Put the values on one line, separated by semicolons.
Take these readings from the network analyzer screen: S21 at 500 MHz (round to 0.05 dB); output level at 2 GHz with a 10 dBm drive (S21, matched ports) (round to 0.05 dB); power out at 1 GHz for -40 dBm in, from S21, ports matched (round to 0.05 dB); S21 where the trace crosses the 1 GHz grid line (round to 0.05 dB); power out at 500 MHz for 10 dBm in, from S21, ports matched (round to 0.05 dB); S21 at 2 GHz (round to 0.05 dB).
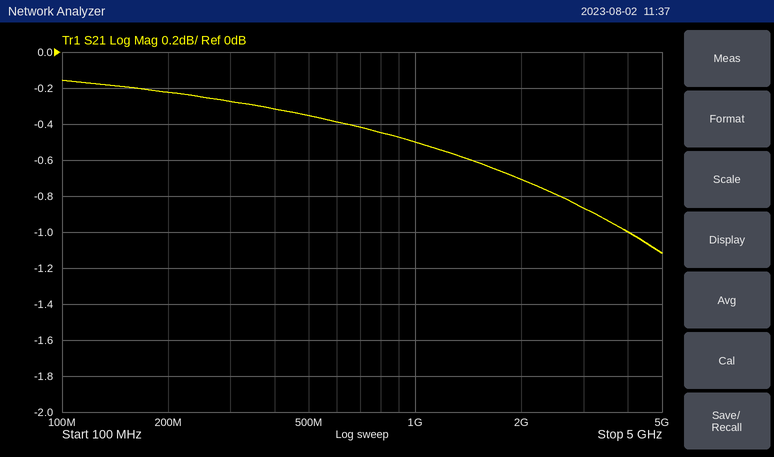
-0.35 dB; 9.30 dBm; -40.50 dBm; -0.50 dB; 9.65 dBm; -0.70 dB
